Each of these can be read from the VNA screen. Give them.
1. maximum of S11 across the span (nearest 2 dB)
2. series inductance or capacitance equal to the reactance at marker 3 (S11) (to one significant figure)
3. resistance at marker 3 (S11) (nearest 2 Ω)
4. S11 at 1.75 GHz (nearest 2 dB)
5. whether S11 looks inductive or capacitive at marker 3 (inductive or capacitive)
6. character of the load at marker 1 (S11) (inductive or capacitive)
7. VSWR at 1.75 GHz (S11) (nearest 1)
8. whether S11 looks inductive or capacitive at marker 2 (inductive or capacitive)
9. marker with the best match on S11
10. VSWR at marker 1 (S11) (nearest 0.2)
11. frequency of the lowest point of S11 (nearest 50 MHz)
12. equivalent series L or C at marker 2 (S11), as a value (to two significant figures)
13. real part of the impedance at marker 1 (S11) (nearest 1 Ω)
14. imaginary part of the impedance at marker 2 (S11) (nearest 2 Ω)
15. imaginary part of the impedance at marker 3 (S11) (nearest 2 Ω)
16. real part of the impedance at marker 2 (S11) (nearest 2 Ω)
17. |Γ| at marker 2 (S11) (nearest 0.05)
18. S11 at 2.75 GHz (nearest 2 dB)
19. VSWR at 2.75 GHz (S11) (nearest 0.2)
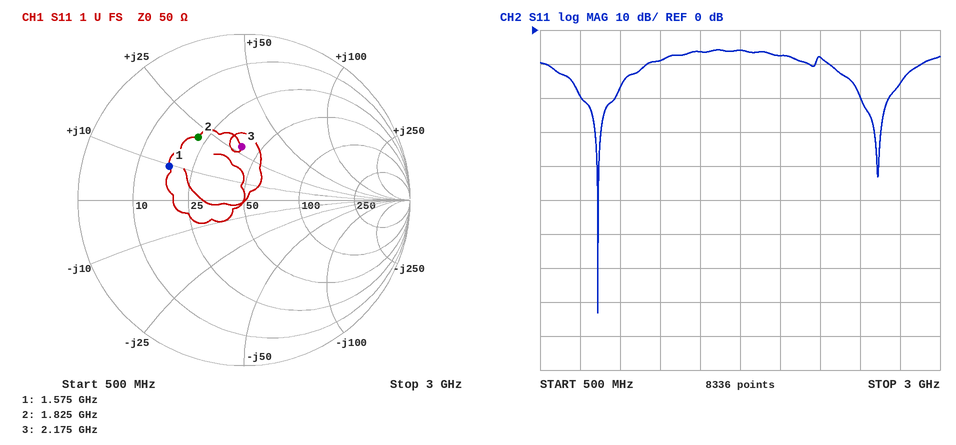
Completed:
-6 dB
2 nH
40 Ω
-6 dB
inductive
inductive
3
inductive
marker 3
3.0
850 MHz
1.9 nH
18 Ω
+22 Ω
+28 Ω
22 Ω
0.45
-16 dB
1.4
